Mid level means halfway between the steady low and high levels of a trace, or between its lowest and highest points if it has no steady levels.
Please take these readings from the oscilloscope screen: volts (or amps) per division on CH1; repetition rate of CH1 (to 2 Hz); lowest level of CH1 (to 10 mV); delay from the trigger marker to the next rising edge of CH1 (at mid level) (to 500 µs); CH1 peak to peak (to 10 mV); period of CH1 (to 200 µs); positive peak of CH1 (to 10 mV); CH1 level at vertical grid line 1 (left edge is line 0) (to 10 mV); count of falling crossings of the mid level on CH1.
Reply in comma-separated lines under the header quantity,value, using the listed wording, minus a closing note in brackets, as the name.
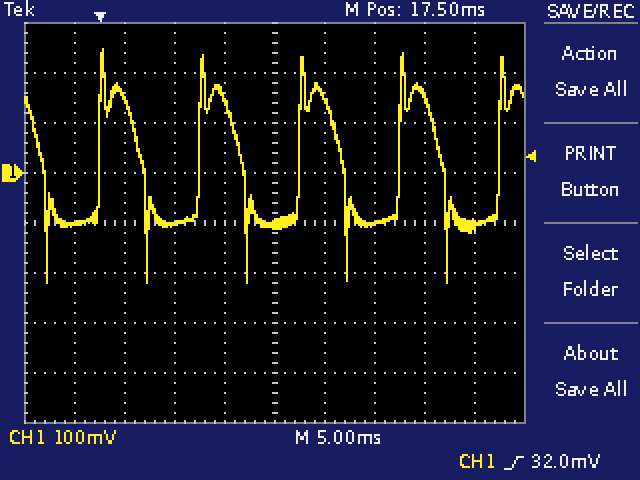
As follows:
quantity,value
volts (or amps) per division on CH1,100 mV
repetition rate of CH1,100 Hz
lowest level of CH1,-220 mV
delay from the trigger marker to the next rising edge of CH1 (at mid level),10.0 ms
CH1 peak to peak,470 mV
period of CH1,10.0 ms
positive peak of CH1,250 mV
CH1 level at vertical grid line 1 (left edge is line 0),-100 mV
count of falling crossings of the mid level on CH1,5
